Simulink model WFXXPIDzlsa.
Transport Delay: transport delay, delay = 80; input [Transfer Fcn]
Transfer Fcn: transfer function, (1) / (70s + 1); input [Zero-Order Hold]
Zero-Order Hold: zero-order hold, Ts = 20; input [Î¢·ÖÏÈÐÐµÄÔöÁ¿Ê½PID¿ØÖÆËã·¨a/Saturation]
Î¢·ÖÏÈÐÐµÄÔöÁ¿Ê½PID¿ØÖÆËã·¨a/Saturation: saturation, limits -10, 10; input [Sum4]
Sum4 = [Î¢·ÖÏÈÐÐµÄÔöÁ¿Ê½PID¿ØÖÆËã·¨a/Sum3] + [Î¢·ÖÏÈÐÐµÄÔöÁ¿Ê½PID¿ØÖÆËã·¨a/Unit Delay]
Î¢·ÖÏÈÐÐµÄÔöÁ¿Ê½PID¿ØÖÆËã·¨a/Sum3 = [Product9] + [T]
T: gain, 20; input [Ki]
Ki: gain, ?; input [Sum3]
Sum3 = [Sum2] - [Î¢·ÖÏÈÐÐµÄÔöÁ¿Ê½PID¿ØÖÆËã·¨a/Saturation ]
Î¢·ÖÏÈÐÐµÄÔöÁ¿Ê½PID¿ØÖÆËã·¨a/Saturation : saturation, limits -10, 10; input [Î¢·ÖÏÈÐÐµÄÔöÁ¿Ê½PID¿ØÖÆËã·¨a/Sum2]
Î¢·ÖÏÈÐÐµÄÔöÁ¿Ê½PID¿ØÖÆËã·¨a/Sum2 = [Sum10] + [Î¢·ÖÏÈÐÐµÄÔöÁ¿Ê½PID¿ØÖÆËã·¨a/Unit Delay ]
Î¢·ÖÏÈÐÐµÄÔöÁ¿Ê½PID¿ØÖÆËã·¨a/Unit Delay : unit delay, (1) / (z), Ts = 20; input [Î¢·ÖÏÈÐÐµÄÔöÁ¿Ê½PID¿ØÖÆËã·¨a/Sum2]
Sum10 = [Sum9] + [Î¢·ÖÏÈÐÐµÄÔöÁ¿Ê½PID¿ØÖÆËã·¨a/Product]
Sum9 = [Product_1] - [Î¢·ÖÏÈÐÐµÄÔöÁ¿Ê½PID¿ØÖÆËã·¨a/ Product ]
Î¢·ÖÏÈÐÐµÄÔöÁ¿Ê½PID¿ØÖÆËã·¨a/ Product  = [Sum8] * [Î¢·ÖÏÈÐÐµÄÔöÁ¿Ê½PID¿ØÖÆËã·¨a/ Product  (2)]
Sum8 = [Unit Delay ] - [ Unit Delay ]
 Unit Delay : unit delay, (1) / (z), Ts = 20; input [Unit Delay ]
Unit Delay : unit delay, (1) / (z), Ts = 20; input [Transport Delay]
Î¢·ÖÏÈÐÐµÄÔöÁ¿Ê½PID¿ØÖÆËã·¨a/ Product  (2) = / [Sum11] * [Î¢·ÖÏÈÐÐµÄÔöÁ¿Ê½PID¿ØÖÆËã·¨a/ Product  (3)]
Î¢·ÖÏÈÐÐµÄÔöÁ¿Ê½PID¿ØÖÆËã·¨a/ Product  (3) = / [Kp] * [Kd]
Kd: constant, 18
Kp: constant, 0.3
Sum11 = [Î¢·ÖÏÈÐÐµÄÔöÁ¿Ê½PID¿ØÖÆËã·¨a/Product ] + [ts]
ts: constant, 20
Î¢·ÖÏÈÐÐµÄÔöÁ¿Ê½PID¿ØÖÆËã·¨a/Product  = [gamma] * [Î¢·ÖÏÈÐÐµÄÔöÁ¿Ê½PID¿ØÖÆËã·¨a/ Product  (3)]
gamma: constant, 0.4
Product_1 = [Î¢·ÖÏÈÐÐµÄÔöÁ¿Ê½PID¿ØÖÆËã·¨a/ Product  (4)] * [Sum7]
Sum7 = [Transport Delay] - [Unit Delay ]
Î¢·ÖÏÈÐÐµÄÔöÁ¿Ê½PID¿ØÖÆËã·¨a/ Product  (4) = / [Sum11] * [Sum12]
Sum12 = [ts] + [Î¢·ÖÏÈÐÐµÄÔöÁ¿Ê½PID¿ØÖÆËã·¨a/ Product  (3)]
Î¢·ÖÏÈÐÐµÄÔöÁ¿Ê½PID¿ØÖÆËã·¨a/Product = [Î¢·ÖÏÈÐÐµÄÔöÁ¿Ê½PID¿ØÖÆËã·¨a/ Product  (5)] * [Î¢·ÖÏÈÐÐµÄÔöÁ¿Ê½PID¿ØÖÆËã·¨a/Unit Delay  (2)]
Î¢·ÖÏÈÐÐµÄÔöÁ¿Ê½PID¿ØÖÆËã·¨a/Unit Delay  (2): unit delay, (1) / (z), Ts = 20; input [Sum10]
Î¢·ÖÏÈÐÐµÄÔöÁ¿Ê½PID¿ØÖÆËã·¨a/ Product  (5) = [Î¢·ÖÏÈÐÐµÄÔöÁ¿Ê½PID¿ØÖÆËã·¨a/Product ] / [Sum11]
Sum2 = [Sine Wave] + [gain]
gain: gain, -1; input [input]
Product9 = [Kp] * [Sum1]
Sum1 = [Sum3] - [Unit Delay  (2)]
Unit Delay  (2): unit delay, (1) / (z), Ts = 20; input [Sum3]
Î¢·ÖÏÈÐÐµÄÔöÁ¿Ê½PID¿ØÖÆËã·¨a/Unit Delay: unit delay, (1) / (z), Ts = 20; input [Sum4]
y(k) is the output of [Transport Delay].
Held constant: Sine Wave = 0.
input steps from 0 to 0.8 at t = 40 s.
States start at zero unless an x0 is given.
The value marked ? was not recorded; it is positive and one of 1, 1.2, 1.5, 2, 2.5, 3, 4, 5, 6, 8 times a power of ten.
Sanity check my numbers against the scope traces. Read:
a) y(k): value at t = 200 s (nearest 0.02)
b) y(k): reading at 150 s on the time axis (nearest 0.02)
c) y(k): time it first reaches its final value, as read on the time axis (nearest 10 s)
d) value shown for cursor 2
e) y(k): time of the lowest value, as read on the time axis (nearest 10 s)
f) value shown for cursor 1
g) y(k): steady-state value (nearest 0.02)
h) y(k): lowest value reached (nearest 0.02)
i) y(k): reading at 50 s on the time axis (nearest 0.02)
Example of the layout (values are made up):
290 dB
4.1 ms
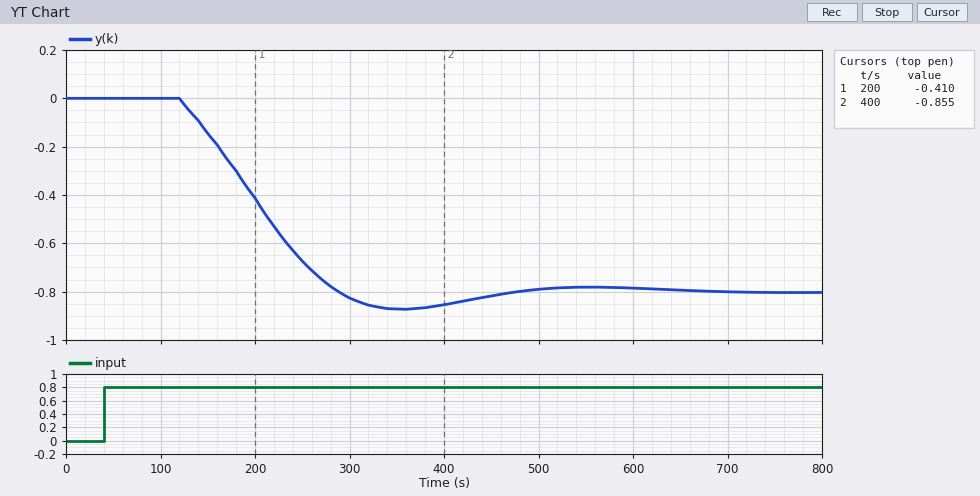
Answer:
-0.42
-0.14
290 s
-0.855
360 s
-0.410
-0.80
-0.88
0.00
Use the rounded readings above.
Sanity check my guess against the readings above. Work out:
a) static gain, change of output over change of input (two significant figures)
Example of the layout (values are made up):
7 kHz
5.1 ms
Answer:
-1.0
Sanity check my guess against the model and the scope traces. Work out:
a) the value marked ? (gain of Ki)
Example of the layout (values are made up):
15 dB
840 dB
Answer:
0.008
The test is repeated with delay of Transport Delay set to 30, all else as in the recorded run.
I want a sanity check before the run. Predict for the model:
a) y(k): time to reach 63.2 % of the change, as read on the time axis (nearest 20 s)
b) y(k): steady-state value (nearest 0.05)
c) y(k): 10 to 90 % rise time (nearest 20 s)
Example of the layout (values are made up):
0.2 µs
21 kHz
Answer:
200 s
-0.80
260 s
